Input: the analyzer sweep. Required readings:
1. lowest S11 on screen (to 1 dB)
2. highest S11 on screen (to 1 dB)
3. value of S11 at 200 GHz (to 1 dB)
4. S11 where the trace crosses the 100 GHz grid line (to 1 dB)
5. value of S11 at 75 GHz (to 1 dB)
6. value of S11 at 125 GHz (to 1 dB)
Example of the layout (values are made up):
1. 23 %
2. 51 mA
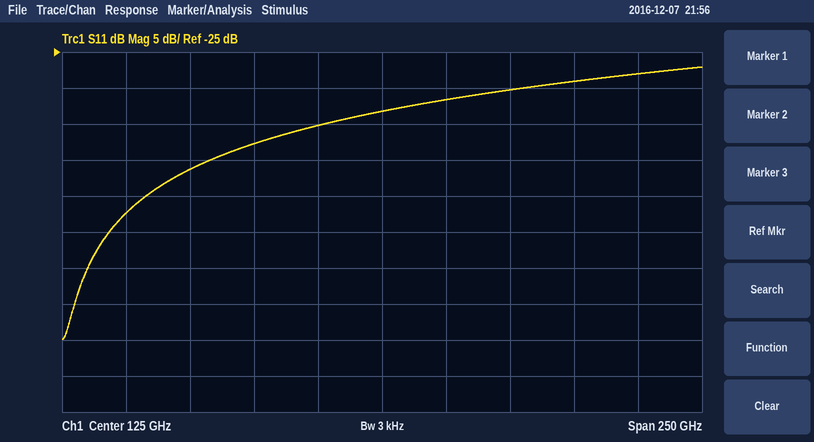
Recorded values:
1. -65 dB
2. -27 dB
3. -29 dB
4. -35 dB
5. -38 dB
6. -33 dB
